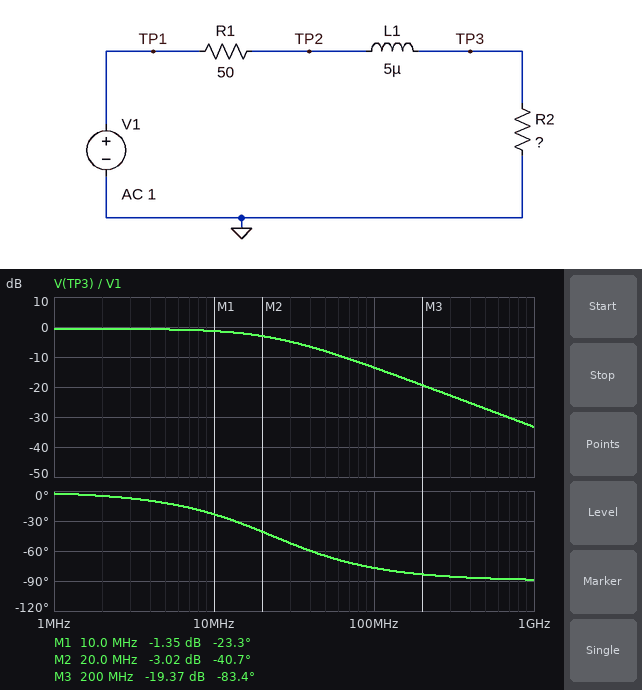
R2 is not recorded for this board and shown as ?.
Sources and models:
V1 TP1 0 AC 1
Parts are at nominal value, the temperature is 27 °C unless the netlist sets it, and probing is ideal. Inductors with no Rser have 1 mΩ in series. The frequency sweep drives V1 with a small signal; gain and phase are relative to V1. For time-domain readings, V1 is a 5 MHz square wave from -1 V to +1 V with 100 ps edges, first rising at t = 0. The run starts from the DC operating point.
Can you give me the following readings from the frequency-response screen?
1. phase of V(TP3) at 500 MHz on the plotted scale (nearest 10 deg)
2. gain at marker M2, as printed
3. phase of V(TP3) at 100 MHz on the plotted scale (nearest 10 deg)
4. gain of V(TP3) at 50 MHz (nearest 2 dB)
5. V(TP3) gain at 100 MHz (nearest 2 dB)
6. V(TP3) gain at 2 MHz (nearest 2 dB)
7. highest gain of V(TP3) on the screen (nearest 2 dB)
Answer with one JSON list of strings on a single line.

["-90 deg", "-3.02 dB", "-80 deg", "-8 dB", "-14 dB", "0 dB", "0 dB"]
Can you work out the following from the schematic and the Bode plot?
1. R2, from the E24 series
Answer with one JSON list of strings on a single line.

["680 Ω"]
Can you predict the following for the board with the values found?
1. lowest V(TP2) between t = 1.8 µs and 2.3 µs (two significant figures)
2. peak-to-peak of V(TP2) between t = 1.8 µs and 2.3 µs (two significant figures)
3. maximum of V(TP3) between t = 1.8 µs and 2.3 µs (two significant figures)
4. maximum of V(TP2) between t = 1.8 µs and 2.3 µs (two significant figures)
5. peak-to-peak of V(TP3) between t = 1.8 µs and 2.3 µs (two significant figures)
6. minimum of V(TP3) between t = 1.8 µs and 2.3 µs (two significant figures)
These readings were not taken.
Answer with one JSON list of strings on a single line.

["-1.1 V", "2.1 V", "930 mV", "1.1 V", "1.9 V", "-930 mV"]
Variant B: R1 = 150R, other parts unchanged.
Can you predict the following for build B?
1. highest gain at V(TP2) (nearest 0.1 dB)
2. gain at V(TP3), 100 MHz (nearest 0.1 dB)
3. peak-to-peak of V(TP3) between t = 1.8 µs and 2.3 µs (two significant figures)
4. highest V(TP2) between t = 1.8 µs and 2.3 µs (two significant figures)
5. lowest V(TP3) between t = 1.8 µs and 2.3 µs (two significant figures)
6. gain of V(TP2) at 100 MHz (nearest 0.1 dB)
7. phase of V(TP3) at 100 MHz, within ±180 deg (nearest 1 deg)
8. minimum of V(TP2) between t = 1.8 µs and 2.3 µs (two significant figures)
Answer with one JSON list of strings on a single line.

["0 dB", "-13.6 dB", "1.6 V", "1.2 V", "-820 mV", "-0.1 dB", "-75 deg", "-1.2 V"]
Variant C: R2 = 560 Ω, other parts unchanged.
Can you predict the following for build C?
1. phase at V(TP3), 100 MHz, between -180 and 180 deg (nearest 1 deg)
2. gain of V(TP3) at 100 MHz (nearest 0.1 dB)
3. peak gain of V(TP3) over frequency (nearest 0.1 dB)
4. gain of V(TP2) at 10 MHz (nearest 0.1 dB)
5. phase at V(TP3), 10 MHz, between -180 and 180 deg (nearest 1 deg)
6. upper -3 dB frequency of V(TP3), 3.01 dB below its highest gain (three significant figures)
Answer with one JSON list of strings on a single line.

["-79 deg", "-15.1 dB", "-0.7 dB", "-0.6 dB", "-27 deg", "19.4 MHz"]
